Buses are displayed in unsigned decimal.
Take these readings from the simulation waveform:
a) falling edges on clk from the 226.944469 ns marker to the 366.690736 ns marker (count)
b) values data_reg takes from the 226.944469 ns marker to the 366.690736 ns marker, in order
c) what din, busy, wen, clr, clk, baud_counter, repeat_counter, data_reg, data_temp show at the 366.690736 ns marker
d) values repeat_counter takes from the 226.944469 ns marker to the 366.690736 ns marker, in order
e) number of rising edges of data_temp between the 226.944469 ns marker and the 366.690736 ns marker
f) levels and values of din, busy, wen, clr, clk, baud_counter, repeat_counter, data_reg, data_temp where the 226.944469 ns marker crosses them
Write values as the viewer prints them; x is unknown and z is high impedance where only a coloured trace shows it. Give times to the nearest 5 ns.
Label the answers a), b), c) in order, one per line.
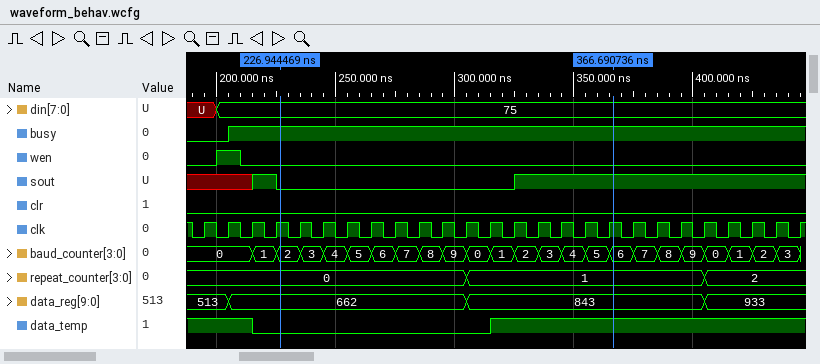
a) 14
b) 662, 843
c) din=75, busy=1, wen=0, clr=0, clk=1, baud_counter=6, repeat_counter=1, data_reg=843, data_temp=1
d) 0, 1
e) 1
f) din=75, busy=1, wen=0, clr=0, clk=1, baud_counter=2, repeat_counter=0, data_reg=662, data_temp=0
